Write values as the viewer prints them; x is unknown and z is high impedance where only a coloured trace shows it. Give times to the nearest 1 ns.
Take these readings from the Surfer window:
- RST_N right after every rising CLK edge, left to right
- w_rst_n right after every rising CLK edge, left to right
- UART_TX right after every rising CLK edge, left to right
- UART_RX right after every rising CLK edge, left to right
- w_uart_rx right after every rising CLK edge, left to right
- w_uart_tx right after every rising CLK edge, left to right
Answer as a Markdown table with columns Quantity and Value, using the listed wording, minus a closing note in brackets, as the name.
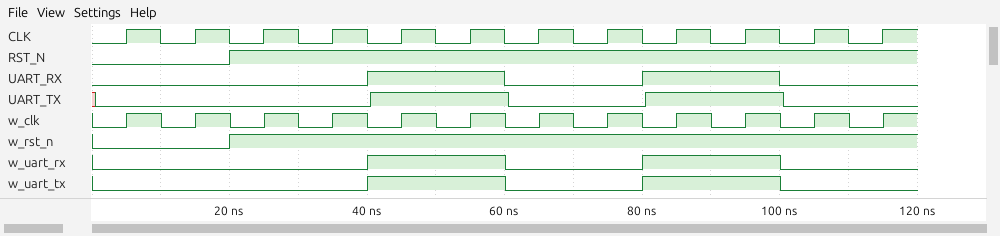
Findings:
| Quantity | Value |
|---|---|
| RST_N right after every rising CLK edge, left to right | 0 0 1 1 1 1 1 1 1 1 1 1 |
| w_rst_n right after every rising CLK edge, left to right | 0 0 1 1 1 1 1 1 1 1 1 1 |
| UART_TX right after every rising CLK edge, left to right | 0 0 0 0 1 1 0 0 1 1 0 0 |
| UART_RX right after every rising CLK edge, left to right | 0 0 0 0 1 1 0 0 1 1 0 0 |
| w_uart_rx right after every rising CLK edge, left to right | 0 0 0 0 1 1 0 0 1 1 0 0 |
| w_uart_tx right after every rising CLK edge, left to right | 0 0 0 0 1 1 0 0 1 1 0 0 |
